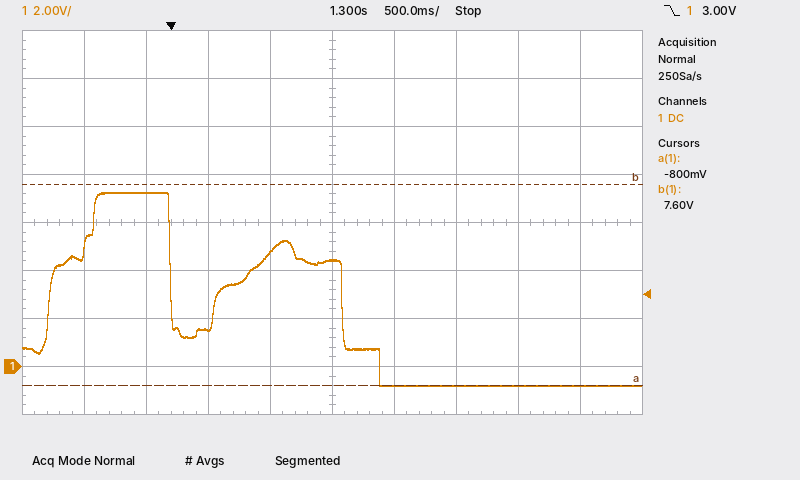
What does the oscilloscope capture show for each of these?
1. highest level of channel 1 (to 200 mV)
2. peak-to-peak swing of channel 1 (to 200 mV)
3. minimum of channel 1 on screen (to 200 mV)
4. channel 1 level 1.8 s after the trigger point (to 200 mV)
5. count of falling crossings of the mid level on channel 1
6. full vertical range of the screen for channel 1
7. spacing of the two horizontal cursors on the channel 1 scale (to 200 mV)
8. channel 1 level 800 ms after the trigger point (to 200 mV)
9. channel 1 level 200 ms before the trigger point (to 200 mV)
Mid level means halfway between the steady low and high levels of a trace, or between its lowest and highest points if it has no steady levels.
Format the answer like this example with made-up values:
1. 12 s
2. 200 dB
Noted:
1. 7.2 V
2. 8.0 V
3. -800 mV
4. -800 mV
5. 2
6. 16 V
7. 8.4 V
8. 4.8 V
9. 7.2 V
